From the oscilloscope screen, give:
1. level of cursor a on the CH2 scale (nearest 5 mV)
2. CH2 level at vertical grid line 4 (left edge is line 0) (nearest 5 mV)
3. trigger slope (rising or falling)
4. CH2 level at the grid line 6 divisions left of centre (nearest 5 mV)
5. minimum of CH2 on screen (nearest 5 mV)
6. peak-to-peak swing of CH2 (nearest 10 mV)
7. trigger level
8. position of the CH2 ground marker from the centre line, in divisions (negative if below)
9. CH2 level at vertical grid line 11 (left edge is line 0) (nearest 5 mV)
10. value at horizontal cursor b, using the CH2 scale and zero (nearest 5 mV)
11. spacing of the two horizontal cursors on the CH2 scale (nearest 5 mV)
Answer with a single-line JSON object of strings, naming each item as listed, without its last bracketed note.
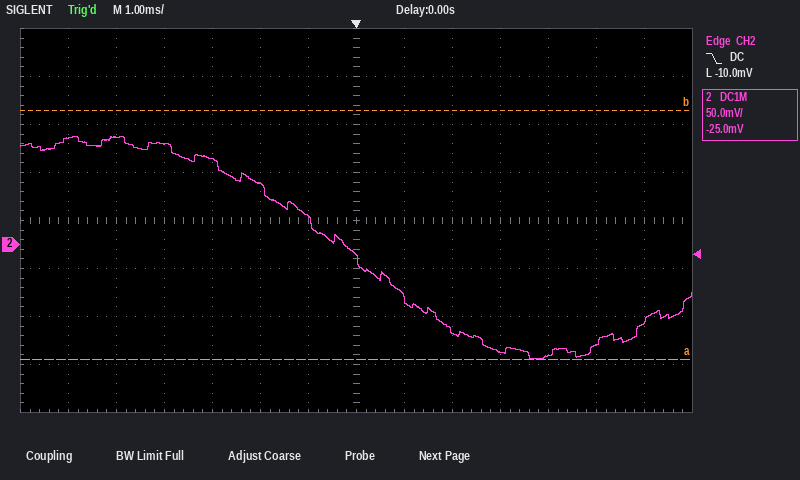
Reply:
{"level of cursor a on the CH2 scale": "-120 mV", "CH2 level at vertical grid line 4 (left edge is line 0)": "90 mV", "trigger slope": "falling", "CH2 level at the grid line 6 divisions left of centre": "110 mV", "minimum of CH2 on screen": "-120 mV", "peak-to-peak swing of CH2": "230 mV", "trigger level": "-10.0 mV", "position of the CH2 ground marker from the centre line, in divisions": "-0.5 div", "CH2 level at vertical grid line 11 (left edge is line 0)": "-115 mV", "value at horizontal cursor b, using the CH2 scale and zero": "140 mV", "spacing of the two horizontal cursors on the CH2 scale": "260 mV"}
